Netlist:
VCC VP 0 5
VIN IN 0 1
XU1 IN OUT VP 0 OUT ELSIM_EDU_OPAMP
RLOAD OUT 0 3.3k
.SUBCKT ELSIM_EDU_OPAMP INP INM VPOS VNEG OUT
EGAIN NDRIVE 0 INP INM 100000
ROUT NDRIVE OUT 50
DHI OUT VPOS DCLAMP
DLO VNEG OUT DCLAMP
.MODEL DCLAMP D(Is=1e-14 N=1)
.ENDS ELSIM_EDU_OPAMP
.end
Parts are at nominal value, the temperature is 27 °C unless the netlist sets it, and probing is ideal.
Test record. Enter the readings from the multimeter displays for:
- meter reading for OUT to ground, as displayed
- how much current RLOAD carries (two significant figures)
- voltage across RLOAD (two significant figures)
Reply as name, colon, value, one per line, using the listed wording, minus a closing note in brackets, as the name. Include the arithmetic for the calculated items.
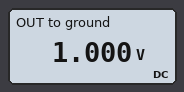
meter reading for OUT to ground, as displayed: 1.000 V
how much current RLOAD carries: (1 V) / 3.3 kΩ = 300 µA
voltage across RLOAD: 1 V = 1.0 V
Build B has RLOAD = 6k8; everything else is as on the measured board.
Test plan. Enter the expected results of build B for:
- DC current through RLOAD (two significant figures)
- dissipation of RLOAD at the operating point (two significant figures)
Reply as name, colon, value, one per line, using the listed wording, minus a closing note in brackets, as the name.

DC current through RLOAD: 150 µA
dissipation of RLOAD at the operating point: 150 µW
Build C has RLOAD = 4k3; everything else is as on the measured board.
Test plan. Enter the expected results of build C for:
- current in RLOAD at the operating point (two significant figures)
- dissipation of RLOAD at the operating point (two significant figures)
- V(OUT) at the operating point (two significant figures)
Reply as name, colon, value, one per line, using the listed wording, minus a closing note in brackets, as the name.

current in RLOAD at the operating point: 230 µA
dissipation of RLOAD at the operating point: 230 µW
V(OUT) at the operating point: 1.0 V
